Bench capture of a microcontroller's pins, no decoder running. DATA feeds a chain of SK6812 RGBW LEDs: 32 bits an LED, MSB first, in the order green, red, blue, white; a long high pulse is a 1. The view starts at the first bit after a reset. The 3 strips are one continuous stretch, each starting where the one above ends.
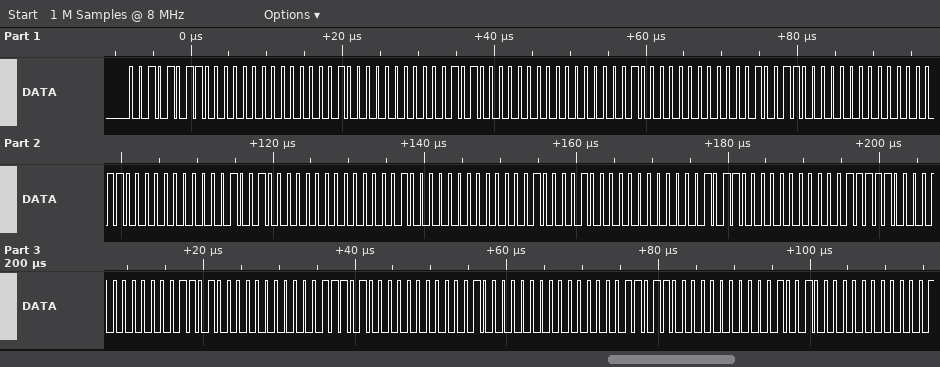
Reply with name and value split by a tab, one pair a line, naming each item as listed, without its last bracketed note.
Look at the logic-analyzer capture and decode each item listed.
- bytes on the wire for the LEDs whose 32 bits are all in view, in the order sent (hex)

bytes on the wire for the LEDs whose 32 bits are all in view, in the order sent	2B 00 02 00 28 00 04 00 26 00 06 00 24 00 08 00 21 00 0B 00 1F 00 0D 00 1D 00 10 00 1B 00 12 00
